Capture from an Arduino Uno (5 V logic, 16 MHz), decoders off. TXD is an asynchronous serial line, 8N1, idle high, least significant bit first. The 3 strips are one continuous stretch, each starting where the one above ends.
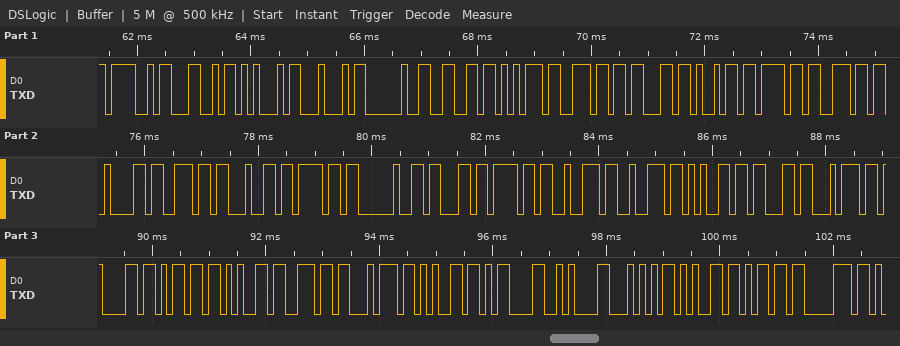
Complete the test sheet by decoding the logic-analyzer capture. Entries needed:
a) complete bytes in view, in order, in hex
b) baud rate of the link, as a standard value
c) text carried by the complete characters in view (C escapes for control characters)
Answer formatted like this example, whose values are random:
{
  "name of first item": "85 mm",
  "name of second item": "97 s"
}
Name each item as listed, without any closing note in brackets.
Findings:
{
  "complete bytes in view, in order, in hex": "4F 4C 45 44 20 66 75 6E 63 69 6F 6E 61 6E 64 6F 20 63 6F 72 72 65 63 74 61 6D 65 6E 74 65 0D 0A 54 65 6D 70",
  "baud rate of the link, as a standard value": "9600 baud",
  "text carried by the complete characters in view": "\"OLED funcionando correctamente\\r\\nTemp\""
}
